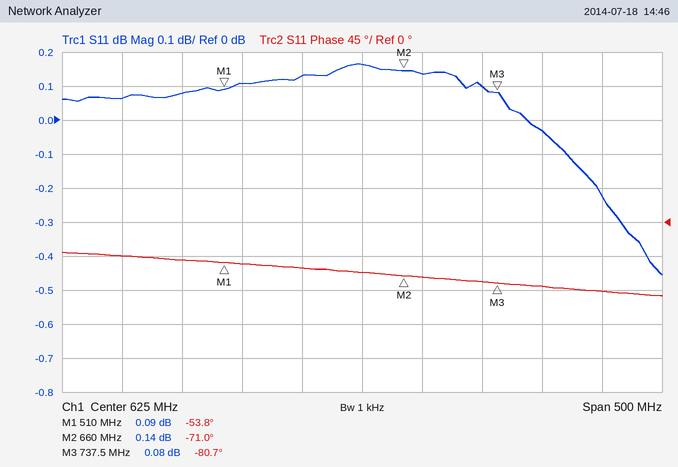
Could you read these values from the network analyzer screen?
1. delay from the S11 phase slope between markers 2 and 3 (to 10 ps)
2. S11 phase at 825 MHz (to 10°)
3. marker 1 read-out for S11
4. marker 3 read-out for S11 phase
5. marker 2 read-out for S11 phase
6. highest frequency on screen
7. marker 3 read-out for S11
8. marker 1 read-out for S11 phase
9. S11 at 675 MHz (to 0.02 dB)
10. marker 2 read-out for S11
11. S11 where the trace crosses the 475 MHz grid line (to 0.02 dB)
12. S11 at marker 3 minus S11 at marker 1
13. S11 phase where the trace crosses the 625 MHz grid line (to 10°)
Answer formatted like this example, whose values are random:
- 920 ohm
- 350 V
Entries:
- 350 ps
- -90°
- 0.09 dB
- -80.7°
- -71.0°
- 875 MHz
- 0.08 dB
- -53.8°
- 0.14 dB
- 0.14 dB
- 0.08 dB
- -0.01 dB
- -70°
